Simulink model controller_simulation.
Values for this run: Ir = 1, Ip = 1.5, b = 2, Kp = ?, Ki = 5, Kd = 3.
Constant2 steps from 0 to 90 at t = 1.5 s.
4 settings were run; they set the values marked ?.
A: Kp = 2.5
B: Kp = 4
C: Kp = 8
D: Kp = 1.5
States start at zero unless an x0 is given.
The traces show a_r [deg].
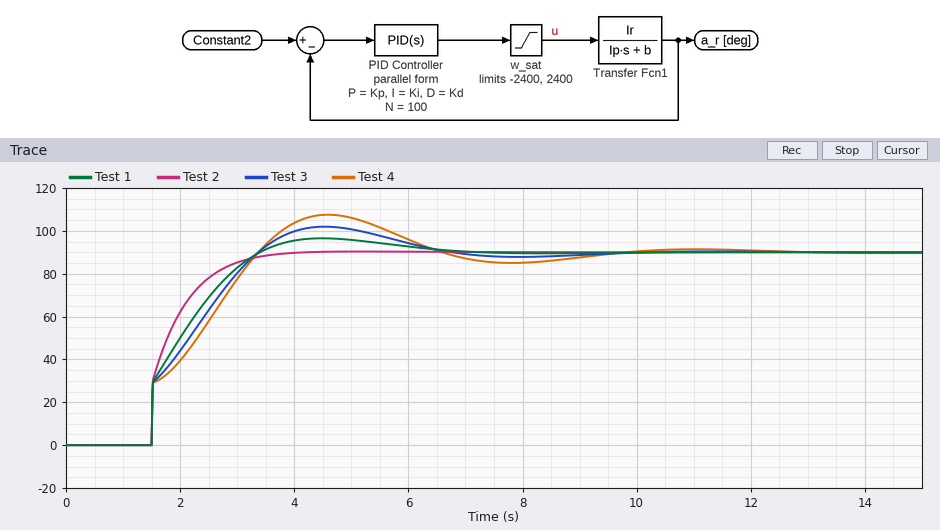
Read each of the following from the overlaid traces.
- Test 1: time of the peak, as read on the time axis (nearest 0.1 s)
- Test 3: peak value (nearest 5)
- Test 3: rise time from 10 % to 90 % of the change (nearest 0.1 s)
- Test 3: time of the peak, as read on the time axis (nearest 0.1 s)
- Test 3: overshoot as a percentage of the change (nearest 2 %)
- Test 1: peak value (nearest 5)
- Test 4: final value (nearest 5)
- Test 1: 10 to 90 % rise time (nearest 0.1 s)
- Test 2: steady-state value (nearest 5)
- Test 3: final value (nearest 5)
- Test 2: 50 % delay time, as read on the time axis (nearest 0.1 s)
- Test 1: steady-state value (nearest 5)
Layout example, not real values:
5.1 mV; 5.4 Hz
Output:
4.5 s; 100; 1.5 s; 4.5 s; 14 %; 95; 90; 1.4 s; 90; 90; 1.7 s; 90
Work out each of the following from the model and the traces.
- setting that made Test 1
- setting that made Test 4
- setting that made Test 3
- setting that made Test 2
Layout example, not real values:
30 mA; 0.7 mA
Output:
B; D; A; C
